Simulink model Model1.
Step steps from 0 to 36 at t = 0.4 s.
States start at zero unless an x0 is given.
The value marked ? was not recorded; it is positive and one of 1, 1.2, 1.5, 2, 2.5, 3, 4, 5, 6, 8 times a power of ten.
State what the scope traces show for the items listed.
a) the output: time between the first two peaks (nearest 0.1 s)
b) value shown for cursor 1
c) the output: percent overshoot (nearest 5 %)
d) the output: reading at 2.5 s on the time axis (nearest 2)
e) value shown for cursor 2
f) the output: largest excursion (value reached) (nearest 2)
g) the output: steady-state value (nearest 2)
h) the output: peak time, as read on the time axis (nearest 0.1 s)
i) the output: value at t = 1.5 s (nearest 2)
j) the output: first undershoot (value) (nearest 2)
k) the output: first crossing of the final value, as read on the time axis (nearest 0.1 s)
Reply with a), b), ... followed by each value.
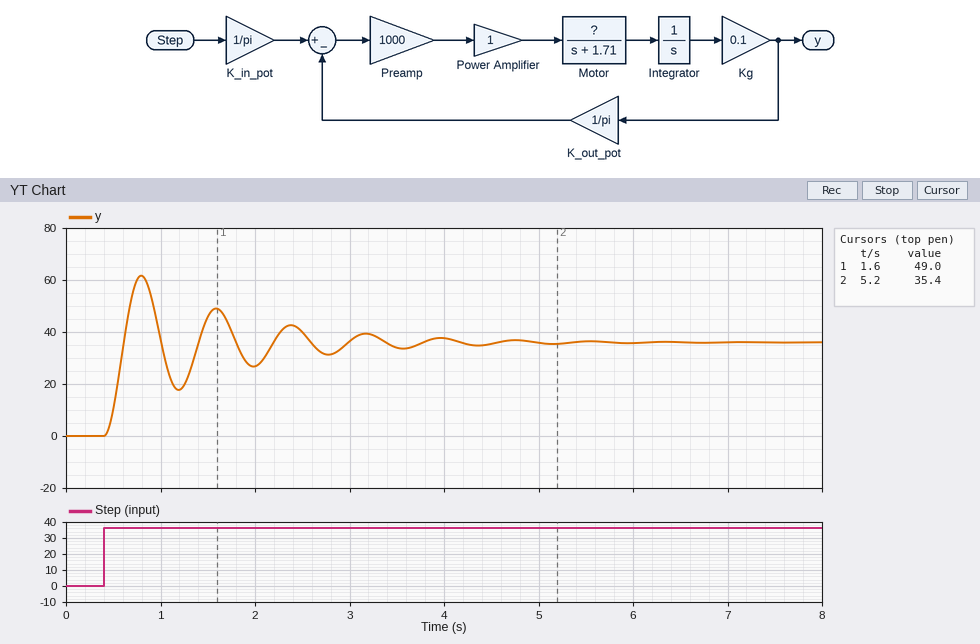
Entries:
a) 0.8 s
b) 49.0
c) 70 %
d) 40
e) 35.4
f) 62
g) 36
h) 0.8 s
i) 46
j) 18
k) 0.6 s
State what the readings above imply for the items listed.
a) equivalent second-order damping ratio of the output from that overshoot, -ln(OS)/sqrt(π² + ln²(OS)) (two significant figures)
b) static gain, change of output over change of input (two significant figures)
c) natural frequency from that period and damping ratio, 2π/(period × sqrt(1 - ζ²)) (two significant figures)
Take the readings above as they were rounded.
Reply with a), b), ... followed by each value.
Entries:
a) 0.11
b) 1.0
c) 7.9 rad/s
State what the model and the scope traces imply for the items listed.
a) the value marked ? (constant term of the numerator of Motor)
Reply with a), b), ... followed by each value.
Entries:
a) 2
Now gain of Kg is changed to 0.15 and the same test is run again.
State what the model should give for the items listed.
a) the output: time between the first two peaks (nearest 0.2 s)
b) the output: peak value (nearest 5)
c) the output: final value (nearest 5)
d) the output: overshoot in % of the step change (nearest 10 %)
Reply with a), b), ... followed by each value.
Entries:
a) 0.6 s
b) 65
c) 35
d) 80 %
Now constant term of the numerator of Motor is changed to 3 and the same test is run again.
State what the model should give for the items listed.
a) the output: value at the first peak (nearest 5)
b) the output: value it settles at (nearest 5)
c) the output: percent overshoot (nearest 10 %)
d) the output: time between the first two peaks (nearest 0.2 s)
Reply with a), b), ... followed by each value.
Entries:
a) 65
b) 35
c) 80 %
d) 0.6 s
